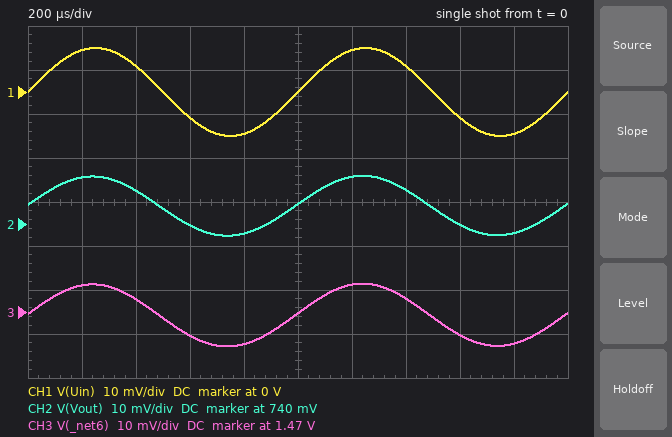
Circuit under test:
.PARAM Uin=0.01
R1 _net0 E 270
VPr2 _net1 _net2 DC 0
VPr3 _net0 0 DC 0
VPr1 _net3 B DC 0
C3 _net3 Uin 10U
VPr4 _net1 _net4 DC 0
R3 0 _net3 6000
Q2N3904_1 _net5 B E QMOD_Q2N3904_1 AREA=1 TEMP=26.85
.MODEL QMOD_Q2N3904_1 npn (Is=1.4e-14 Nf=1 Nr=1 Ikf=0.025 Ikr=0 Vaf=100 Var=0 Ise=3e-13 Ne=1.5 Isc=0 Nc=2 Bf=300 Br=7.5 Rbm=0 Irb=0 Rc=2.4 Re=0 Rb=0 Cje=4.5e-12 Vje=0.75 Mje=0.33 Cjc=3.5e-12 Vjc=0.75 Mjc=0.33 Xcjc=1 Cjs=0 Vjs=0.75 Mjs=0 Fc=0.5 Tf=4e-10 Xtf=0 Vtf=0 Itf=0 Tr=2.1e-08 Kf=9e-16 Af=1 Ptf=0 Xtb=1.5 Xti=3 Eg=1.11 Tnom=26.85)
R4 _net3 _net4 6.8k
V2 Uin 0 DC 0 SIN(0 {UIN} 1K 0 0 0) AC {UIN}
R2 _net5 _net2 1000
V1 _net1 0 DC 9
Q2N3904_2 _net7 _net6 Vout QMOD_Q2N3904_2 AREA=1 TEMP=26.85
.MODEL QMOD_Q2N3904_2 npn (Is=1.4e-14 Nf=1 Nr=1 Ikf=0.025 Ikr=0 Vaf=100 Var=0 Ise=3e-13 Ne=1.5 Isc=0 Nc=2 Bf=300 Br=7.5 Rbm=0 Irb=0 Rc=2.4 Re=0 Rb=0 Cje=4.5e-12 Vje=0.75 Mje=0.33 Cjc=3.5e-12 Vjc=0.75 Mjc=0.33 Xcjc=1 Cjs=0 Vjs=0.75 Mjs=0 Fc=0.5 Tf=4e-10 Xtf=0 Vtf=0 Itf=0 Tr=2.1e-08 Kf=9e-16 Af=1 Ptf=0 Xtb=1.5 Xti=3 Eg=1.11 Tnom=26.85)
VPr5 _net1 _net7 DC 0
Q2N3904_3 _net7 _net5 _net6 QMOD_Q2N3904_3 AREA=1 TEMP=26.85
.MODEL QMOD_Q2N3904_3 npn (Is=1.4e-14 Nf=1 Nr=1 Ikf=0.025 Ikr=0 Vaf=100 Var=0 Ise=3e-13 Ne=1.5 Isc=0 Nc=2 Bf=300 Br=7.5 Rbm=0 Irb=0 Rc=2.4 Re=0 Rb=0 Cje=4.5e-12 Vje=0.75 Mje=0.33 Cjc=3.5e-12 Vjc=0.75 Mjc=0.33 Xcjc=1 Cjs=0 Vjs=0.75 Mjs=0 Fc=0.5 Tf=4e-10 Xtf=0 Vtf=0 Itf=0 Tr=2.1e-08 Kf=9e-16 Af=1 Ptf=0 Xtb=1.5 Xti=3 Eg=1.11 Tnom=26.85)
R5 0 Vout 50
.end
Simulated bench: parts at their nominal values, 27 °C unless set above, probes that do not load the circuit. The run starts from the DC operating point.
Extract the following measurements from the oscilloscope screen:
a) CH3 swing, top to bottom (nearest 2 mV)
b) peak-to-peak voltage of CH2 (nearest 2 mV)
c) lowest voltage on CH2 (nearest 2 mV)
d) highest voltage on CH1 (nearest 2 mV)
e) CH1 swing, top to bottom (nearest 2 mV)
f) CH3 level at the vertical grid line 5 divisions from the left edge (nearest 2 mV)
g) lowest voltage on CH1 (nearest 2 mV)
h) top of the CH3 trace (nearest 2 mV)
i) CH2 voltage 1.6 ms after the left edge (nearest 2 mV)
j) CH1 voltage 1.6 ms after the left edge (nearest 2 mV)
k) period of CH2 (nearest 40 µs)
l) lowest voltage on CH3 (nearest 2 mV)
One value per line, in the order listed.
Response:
14 mV
14 mV
738 mV
10 mV
20 mV
1.470 V
-10 mV
1.476 V
740 mV
-6 mV
1.00 ms
1.462 V
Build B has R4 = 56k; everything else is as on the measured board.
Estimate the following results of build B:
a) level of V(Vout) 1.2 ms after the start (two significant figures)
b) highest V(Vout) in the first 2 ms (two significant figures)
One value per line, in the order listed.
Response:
6.7 V
6.8 V
